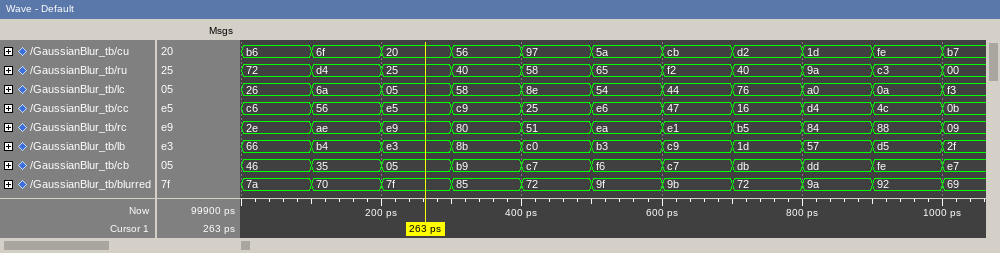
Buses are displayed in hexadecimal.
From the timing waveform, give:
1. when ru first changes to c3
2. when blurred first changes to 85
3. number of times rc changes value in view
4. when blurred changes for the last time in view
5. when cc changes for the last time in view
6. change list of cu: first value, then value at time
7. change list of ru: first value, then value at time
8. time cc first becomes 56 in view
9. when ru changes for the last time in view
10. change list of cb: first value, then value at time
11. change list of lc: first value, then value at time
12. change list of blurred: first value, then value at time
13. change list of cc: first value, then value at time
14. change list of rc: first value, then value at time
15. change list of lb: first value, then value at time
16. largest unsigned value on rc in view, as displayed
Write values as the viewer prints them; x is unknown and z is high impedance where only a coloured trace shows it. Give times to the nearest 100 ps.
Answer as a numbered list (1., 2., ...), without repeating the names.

1. 900 ps
2. 300 ps
3. 10
4. 1000 ps
5. 1000 ps
6. b6, 6f at 100 ps, 20 at 200 ps, 56 at 300 ps, 97 at 400 ps, 5a at 500 ps, cb at 600 ps, d2 at 700 ps, 1d at 800 ps, fe at 900 ps, b7 at 1000 ps
7. 72, d4 at 100 ps, 25 at 200 ps, 40 at 300 ps, 58 at 400 ps, 65 at 500 ps, f2 at 600 ps, 40 at 700 ps, 9a at 800 ps, c3 at 900 ps, 00 at 1000 ps
8. 100 ps
9. 1000 ps
10. 46, 35 at 100 ps, 05 at 200 ps, b9 at 300 ps, c7 at 400 ps, f6 at 500 ps, c7 at 600 ps, db at 700 ps, dd at 800 ps, fe at 900 ps, e7 at 1000 ps
11. 26, 6a at 100 ps, 05 at 200 ps, 58 at 300 ps, 8e at 400 ps, 54 at 500 ps, 44 at 600 ps, 76 at 700 ps, a0 at 800 ps, 0a at 900 ps, f3 at 1000 ps
12. 7a, 70 at 100 ps, 7f at 200 ps, 85 at 300 ps, 72 at 400 ps, 9f at 500 ps, 9b at 600 ps, 72 at 700 ps, 9a at 800 ps, 92 at 900 ps, 69 at 1000 ps
13. c6, 56 at 100 ps, e5 at 200 ps, c9 at 300 ps, 25 at 400 ps, e6 at 500 ps, 47 at 600 ps, 16 at 700 ps, d4 at 800 ps, 4c at 900 ps, 0b at 1000 ps
14. 2e, ae at 100 ps, e9 at 200 ps, 80 at 300 ps, 51 at 400 ps, ea at 500 ps, e1 at 600 ps, b5 at 700 ps, 84 at 800 ps, 88 at 900 ps, 09 at 1000 ps
15. 66, b4 at 100 ps, e3 at 200 ps, 8b at 300 ps, c0 at 400 ps, b3 at 500 ps, c9 at 600 ps, 1d at 700 ps, 57 at 800 ps, d5 at 900 ps, 2f at 1000 ps
16. ea
